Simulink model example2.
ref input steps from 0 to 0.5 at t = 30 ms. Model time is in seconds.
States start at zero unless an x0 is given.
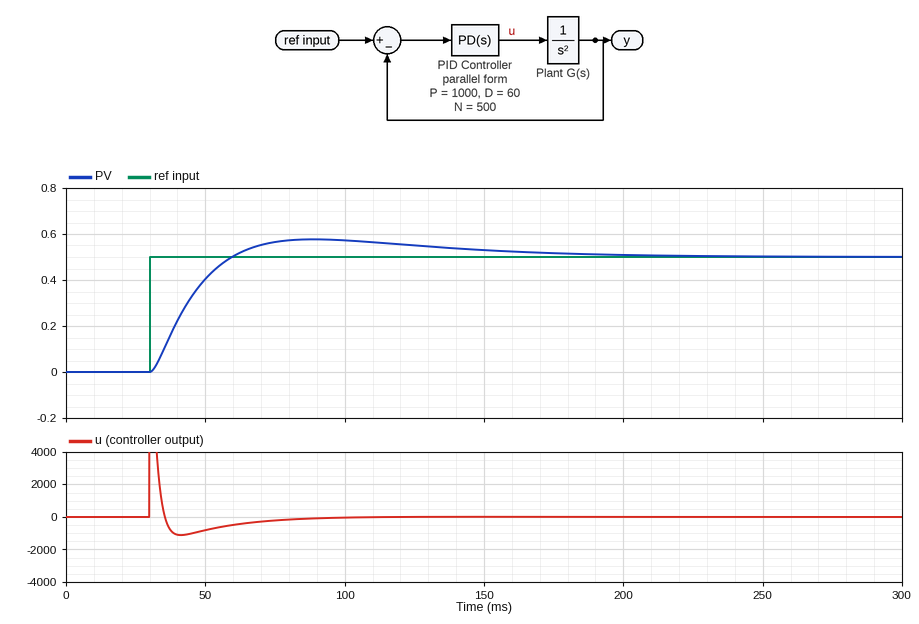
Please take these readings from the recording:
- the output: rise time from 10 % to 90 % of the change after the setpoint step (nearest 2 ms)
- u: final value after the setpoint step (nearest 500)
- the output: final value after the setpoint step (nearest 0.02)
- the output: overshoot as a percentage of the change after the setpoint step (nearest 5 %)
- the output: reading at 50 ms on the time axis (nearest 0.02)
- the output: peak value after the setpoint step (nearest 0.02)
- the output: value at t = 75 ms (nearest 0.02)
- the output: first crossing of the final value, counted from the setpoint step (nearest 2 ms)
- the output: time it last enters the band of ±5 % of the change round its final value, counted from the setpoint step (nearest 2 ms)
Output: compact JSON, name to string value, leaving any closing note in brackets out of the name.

{"the output: rise time from 10 % to 90 % of the change after the setpoint step": "20 ms", "u: final value after the setpoint step": "0", "the output: final value after the setpoint step": "0.50", "the output: overshoot as a percentage of the change after the setpoint step": "15 %", "the output: reading at 50 ms on the time axis": "0.40", "the output: peak value after the setpoint step": "0.58", "the output: value at t = 75 ms": "0.56", "the output: first crossing of the final value, counted from the setpoint step": "30 ms", "the output: time it last enters the band of ±5 % of the change round its final value, counted from the setpoint step": "128 ms"}
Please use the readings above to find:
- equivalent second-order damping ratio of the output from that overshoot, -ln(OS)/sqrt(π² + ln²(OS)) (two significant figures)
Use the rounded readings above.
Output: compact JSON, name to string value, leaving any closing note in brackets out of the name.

{"equivalent second-order damping ratio of the output from that overshoot, -ln(OS)/sqrt(π² + ln²(OS))": "0.52"}
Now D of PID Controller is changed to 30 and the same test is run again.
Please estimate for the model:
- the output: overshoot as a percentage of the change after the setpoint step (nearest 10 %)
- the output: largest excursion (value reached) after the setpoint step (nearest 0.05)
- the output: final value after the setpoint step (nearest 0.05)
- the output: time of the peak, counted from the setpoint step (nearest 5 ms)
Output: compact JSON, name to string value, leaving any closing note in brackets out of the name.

{"the output: overshoot as a percentage of the change after the setpoint step": "30 %", "the output: largest excursion (value reached) after the setpoint step": "0.65", "the output: final value after the setpoint step": "0.50", "the output: time of the peak, counted from the setpoint step": "75 ms"}
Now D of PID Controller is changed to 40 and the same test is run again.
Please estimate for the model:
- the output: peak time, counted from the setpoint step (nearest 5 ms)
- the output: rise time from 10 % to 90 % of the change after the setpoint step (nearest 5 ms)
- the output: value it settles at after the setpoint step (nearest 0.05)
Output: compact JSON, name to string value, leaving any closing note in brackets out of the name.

{"the output: peak time, counted from the setpoint step": "70 ms", "the output: rise time from 10 % to 90 % of the change after the setpoint step": "25 ms", "the output: value it settles at after the setpoint step": "0.50"}
